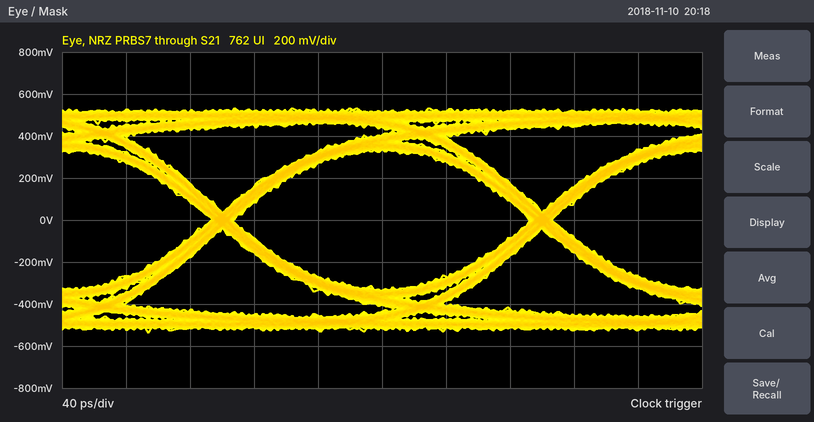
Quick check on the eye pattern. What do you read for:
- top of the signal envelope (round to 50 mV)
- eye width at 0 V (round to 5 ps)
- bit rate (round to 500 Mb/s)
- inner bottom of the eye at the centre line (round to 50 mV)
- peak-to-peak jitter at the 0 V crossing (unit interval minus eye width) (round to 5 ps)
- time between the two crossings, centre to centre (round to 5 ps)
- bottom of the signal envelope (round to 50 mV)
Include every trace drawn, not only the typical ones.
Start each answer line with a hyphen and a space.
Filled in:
- 550 mV
- 185 ps
- 5.0 Gb/s
- -350 mV
- 15 ps
- 200 ps
- -550 mV
